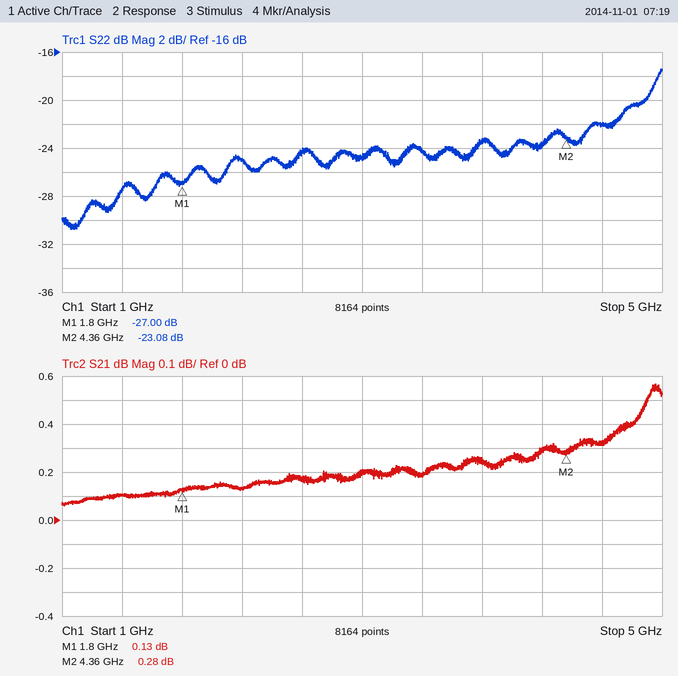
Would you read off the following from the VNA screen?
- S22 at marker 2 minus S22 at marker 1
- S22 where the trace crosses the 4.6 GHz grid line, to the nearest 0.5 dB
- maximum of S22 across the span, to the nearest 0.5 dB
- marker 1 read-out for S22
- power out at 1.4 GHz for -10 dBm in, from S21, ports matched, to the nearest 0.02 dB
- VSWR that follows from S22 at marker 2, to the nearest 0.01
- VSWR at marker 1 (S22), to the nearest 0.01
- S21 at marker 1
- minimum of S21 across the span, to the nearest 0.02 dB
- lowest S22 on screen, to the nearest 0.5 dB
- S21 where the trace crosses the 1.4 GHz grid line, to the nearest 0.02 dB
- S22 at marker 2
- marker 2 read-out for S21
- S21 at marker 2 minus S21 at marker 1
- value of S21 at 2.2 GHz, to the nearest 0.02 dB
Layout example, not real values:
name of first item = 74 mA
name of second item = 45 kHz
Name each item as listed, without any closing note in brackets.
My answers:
S22 at marker 2 minus S22 at marker 1 = 3.92 dB
S22 where the trace crosses the 4.6 GHz grid line, to the nearest 0.5 dB = -22.0 dB
maximum of S22 across the span, to the nearest 0.5 dB = -17.5 dB
marker 1 read-out for S22 = -27.00 dB
power out at 1.4 GHz for -10 dBm in, from S21, ports matched, to the nearest 0.02 dB = -9.90 dBm
VSWR that follows from S22 at marker 2, to the nearest 0.01 = 1.15
VSWR at marker 1 (S22), to the nearest 0.01 = 1.09
S21 at marker 1 = 0.13 dB
minimum of S21 across the span, to the nearest 0.02 dB = 0.06 dB
lowest S22 on screen, to the nearest 0.5 dB = -31.0 dB
S21 where the trace crosses the 1.4 GHz grid line, to the nearest 0.02 dB = 0.10 dB
S22 at marker 2 = -23.08 dB
marker 2 read-out for S21 = 0.28 dB
S21 at marker 2 minus S21 at marker 1 = 0.15 dB
value of S21 at 2.2 GHz, to the nearest 0.02 dB = 0.14 dB
